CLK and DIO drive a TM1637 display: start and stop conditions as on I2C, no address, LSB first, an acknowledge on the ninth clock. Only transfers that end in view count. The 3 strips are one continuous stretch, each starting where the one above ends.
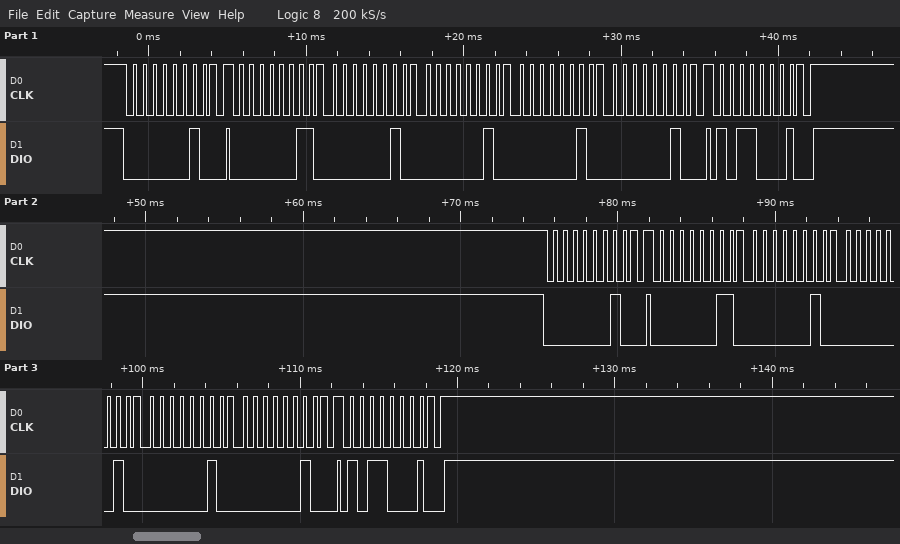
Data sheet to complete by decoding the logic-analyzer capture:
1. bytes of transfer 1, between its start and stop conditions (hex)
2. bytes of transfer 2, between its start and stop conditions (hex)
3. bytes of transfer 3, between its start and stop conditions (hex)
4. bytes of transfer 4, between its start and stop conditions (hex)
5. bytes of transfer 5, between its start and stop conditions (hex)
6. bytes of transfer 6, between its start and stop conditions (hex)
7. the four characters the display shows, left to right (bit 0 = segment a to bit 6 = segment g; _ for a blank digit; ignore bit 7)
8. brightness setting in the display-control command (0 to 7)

40
C0 40 40 40 40
8D
40
C0 40 40 40 40
8D
----
5
